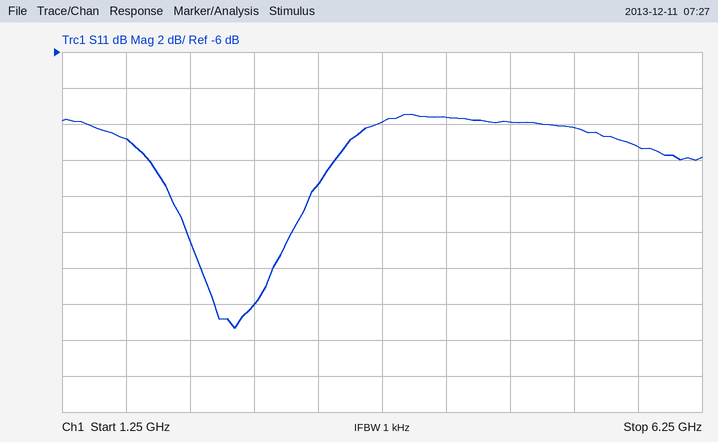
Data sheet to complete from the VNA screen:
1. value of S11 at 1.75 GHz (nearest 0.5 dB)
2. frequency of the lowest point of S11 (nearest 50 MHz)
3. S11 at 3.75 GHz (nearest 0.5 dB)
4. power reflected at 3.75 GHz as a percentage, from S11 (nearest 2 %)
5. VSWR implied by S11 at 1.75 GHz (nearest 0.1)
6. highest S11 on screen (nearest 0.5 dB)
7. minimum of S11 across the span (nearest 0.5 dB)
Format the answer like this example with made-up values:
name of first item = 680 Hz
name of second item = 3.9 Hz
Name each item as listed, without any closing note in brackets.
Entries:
value of S11 at 1.75 GHz = -11.0 dB
frequency of the lowest point of S11 = 2.60 GHz
S11 at 3.75 GHz = -10.0 dB
power reflected at 3.75 GHz as a percentage, from S11 = 10 %
VSWR implied by S11 at 1.75 GHz = 1.8
highest S11 on screen = -9.5 dB
minimum of S11 across the span = -21.5 dB
